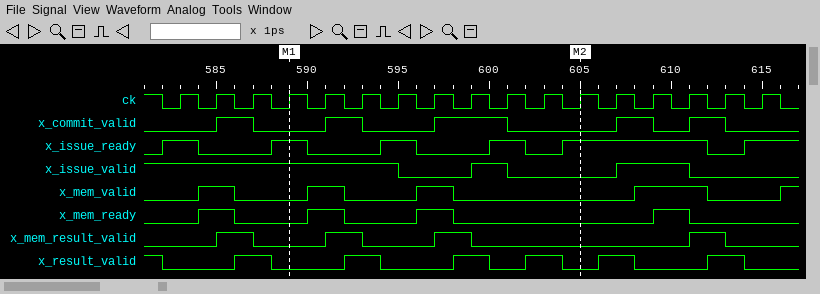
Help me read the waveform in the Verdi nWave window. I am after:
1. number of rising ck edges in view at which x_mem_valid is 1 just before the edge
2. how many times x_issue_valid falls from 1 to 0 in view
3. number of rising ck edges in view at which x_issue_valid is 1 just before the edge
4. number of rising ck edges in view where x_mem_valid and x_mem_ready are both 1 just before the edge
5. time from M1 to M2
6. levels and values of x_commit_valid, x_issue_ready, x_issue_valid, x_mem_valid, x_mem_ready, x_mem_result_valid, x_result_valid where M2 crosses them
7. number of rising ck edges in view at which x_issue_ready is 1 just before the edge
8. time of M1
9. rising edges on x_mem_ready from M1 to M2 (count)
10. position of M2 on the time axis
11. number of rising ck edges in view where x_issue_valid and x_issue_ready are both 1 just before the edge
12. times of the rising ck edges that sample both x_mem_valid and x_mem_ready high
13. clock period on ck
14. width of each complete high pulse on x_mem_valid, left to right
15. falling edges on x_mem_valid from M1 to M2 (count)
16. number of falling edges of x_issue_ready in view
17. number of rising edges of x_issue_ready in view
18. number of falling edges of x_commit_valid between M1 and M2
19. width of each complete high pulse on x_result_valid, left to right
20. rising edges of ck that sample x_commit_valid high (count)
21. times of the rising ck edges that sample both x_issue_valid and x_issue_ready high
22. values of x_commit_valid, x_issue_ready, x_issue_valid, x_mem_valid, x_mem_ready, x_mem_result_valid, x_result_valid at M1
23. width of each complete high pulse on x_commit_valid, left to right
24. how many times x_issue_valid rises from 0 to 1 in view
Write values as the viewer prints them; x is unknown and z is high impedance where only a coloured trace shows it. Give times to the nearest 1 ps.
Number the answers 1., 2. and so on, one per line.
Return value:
1. 5
2. 3
3. 10
4. 4
5. 16 ps
6. x_commit_valid=0, x_issue_ready=1, x_issue_valid=0, x_mem_valid=0, x_mem_ready=0, x_mem_result_valid=0, x_result_valid=0
7. 9
8. 589 ps
9. 2
10. 605 ps
11. 6
12. 585 ps, 591 ps, 597 ps, 611 ps
13. 2 ps
14. 2 ps, 2 ps, 2 ps, 4 ps
15. 2
16. 5
17. 6
18. 2
19. 2 ps, 2 ps, 2 ps, 2 ps, 2 ps, 2 ps
20. 6
21. 583 ps, 589 ps, 595 ps, 601 ps, 609 ps, 611 ps
22. x_commit_valid=0, x_issue_ready=1, x_issue_valid=1, x_mem_valid=0, x_mem_ready=0, x_mem_result_valid=0, x_result_valid=0
23. 2 ps, 2 ps, 4 ps, 2 ps, 2 ps
24. 2
